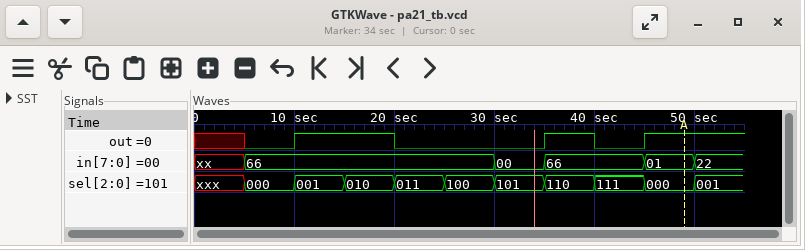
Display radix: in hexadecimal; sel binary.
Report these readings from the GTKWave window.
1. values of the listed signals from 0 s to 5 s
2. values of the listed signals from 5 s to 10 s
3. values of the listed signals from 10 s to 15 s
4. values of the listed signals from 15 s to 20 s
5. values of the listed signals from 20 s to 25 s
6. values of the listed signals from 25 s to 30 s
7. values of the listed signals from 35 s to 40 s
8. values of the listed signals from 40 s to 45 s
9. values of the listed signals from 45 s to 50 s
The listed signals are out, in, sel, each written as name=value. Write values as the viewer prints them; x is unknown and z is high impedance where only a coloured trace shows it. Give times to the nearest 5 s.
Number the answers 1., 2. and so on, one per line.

1. out=x, in=xx, sel=xxx
2. out=0, in=66, sel=000
3. out=1, in=66, sel=001
4. out=1, in=66, sel=010
5. out=0, in=66, sel=011
6. out=0, in=66, sel=100
7. out=1, in=66, sel=110
8. out=0, in=66, sel=111
9. out=1, in=01, sel=000
